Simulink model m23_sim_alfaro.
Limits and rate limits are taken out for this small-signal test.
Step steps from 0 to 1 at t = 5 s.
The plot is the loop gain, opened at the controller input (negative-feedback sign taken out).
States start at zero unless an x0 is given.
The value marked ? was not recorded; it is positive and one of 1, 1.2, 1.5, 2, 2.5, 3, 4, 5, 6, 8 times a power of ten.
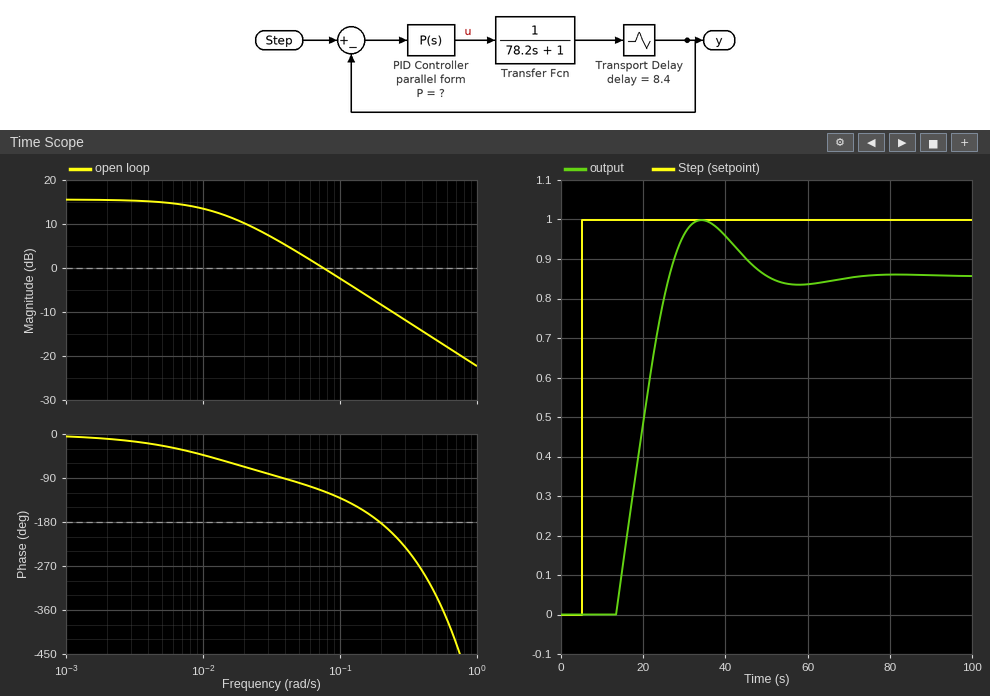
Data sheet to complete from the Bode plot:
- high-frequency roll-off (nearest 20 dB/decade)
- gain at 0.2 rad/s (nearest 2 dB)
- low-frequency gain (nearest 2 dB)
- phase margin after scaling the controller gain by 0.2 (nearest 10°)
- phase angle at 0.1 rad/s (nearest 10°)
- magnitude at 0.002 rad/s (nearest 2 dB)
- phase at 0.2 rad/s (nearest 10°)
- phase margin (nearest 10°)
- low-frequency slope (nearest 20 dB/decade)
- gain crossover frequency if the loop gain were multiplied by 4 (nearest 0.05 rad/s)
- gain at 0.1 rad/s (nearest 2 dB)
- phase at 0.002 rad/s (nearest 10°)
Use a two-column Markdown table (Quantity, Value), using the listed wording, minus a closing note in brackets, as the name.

| Quantity | Value |
|---|---|
| high-frequency roll-off | -20 dB/decade |
| gain at 0.2 rad/s | -8 dB |
| low-frequency gain | 16 dB |
| phase margin after scaling the controller gain by 0.2 | 140° |
| phase angle at 0.1 rad/s | -130° |
| magnitude at 0.002 rad/s | 16 dB |
| phase at 0.2 rad/s | -180° |
| phase margin | 60° |
| low-frequency slope | 0 dB/decade |
| gain crossover frequency if the loop gain were multiplied by 4 | 0.30 rad/s |
| gain at 0.1 rad/s | -2 dB |
| phase at 0.002 rad/s | -10° |
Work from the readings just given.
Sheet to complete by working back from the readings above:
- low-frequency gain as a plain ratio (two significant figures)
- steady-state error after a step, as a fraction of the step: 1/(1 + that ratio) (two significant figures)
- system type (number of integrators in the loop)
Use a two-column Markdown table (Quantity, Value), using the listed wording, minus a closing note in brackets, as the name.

| Quantity | Value |
|---|---|
| low-frequency gain as a plain ratio | 6.3 |
| steady-state error after a step, as a fraction of the step: 1/(1 + that ratio) | 0.14 |
| system type | 0 |
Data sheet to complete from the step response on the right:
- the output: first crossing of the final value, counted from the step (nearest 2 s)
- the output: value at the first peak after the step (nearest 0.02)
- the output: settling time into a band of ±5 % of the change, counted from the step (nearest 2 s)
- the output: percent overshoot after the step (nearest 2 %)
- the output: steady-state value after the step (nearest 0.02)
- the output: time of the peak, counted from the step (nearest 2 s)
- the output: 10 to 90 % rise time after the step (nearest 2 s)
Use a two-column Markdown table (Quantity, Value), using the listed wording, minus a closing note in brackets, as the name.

| Quantity | Value |
|---|---|
| the output: first crossing of the final value, counted from the step | 22 s |
| the output: value at the first peak after the step | 1.00 |
| the output: settling time into a band of ±5 % of the change, counted from the step | 40 s |
| the output: percent overshoot after the step | 16 % |
| the output: steady-state value after the step | 0.86 |
| the output: time of the peak, counted from the step | 30 s |
| the output: 10 to 90 % rise time after the step | 10 s |
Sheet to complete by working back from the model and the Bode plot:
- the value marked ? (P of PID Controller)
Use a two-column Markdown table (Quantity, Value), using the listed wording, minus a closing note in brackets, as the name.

| Quantity | Value |
|---|---|
| the value marked ? | 6 |
